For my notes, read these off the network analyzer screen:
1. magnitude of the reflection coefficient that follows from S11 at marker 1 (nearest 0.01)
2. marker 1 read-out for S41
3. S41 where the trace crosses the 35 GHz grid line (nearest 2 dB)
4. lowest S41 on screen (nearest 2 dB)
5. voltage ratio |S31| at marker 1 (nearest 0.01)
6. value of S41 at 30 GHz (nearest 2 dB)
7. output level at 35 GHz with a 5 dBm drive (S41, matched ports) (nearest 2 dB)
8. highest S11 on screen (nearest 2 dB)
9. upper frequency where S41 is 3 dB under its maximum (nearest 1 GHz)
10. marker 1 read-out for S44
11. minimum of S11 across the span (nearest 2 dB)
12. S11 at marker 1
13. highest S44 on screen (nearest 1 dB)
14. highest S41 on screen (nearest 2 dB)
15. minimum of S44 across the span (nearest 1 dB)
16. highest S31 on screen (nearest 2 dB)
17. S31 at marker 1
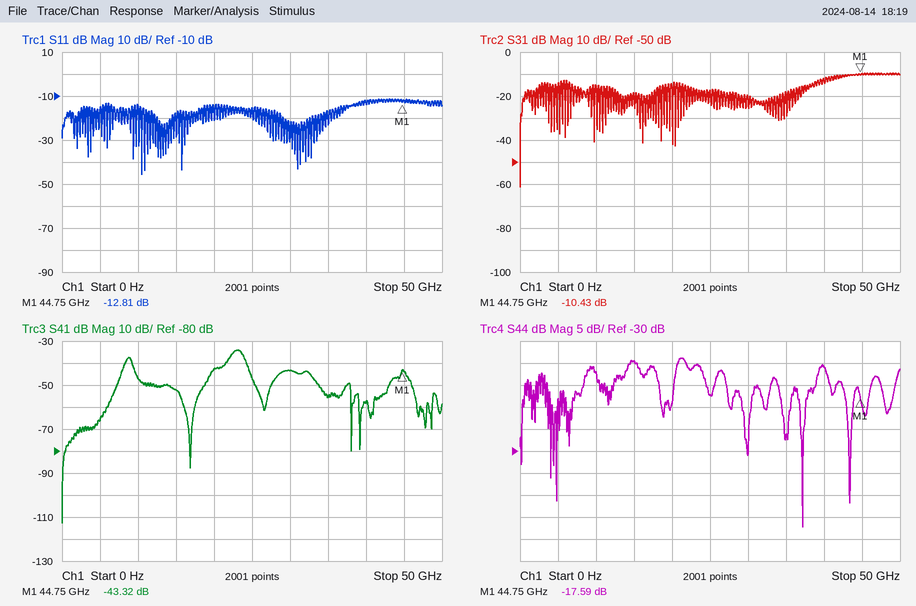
0.23
-43.32 dB
-56 dB
-112 dB
0.30
-44 dB
-50 dBm
-12 dB
24 GHz
-17.59 dB
-46 dB
-12.81 dB
-9 dB
-34 dB
-47 dB
-10 dB
-10.43 dB
